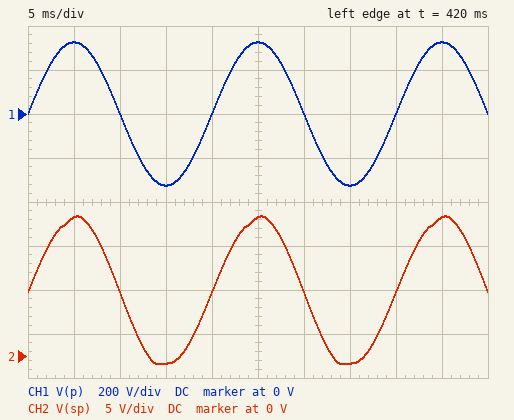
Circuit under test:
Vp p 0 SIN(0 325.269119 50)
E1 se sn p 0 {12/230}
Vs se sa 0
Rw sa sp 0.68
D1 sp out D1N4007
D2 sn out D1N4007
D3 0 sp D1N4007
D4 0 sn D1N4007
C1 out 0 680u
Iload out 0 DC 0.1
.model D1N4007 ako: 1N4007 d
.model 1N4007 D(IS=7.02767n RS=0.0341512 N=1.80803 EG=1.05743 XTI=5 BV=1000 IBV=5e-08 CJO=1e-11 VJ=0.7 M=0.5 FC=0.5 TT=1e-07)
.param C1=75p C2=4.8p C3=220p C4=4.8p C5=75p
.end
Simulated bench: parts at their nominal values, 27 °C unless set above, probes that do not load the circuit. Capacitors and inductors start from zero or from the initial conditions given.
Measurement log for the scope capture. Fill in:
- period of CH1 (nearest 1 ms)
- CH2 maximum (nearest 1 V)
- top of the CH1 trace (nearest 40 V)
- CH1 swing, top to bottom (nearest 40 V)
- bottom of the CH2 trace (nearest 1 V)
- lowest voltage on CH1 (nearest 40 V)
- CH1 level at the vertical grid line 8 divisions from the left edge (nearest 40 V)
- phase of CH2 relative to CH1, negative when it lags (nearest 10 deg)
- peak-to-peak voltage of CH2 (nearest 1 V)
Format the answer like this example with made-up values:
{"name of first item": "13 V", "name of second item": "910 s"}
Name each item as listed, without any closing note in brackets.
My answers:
{"period of CH1": "20 ms", "CH2 maximum": "16 V", "top of the CH1 trace": "320 V", "CH1 swing, top to bottom": "640 V", "bottom of the CH2 trace": "-1 V", "lowest voltage on CH1": "-320 V", "CH1 level at the vertical grid line 8 divisions from the left edge": "0 V", "phase of CH2 relative to CH1, negative when it lags": "0 deg", "peak-to-peak voltage of CH2": "17 V"}
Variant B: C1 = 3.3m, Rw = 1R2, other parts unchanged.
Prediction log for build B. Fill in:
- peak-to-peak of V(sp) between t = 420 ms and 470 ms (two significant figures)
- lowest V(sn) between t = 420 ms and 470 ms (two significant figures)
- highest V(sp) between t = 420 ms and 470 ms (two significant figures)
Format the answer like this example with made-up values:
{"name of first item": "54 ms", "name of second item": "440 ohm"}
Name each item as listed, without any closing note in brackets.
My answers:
{"peak-to-peak of V(sp) between t = 420 ms and 470 ms": "16 V", "lowest V(sn) between t = 420 ms and 470 ms": "-880 mV", "highest V(sp) between t = 420 ms and 470 ms": "15 V"}
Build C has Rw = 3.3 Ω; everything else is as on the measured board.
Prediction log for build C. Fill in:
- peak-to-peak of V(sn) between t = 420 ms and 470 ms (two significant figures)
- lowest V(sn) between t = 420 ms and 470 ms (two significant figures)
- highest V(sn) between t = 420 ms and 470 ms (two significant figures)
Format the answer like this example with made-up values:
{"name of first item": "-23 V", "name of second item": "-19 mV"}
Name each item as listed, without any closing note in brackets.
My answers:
{"peak-to-peak of V(sn) between t = 420 ms and 470 ms": "16 V", "lowest V(sn) between t = 420 ms and 470 ms": "-860 mV", "highest V(sn) between t = 420 ms and 470 ms": "15 V"}
